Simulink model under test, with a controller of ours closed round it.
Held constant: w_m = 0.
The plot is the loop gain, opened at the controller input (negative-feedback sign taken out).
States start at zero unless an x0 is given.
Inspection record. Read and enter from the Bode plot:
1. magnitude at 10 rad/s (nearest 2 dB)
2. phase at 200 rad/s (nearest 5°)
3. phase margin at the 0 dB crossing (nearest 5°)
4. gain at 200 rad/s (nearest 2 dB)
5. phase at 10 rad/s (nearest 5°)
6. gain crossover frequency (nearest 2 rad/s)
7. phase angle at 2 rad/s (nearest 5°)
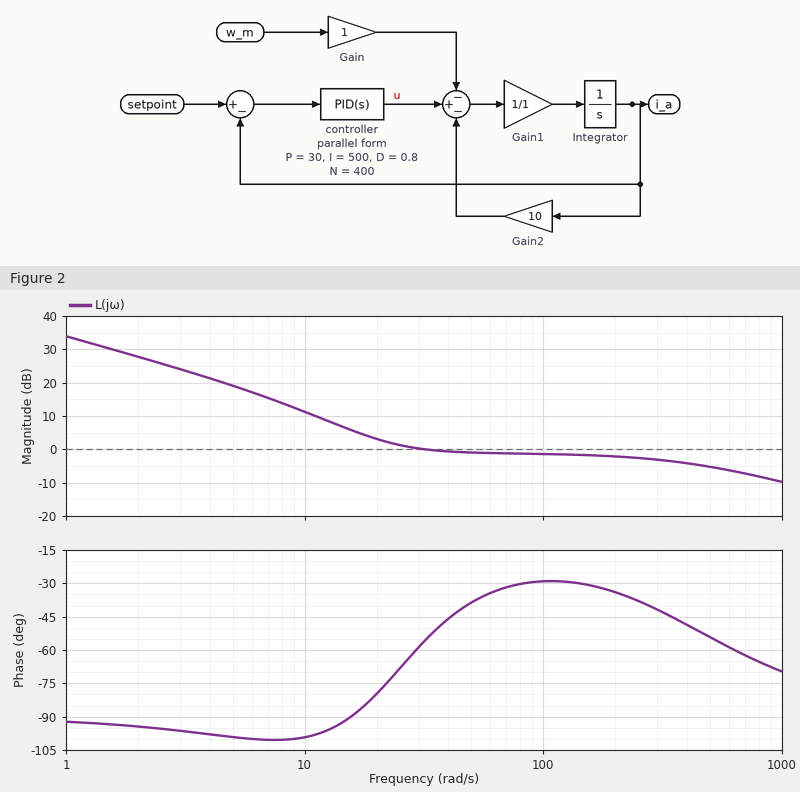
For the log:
12 dB
-35°
125°
-2 dB
-100°
32 rad/s
-95°
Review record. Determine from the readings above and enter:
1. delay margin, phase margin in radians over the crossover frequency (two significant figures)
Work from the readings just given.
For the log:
0.068 s
